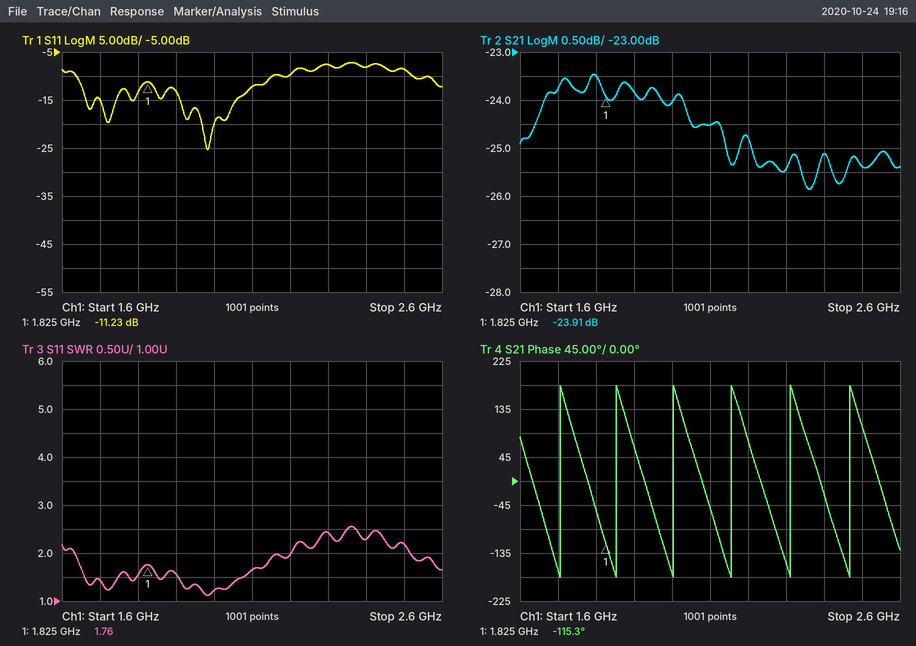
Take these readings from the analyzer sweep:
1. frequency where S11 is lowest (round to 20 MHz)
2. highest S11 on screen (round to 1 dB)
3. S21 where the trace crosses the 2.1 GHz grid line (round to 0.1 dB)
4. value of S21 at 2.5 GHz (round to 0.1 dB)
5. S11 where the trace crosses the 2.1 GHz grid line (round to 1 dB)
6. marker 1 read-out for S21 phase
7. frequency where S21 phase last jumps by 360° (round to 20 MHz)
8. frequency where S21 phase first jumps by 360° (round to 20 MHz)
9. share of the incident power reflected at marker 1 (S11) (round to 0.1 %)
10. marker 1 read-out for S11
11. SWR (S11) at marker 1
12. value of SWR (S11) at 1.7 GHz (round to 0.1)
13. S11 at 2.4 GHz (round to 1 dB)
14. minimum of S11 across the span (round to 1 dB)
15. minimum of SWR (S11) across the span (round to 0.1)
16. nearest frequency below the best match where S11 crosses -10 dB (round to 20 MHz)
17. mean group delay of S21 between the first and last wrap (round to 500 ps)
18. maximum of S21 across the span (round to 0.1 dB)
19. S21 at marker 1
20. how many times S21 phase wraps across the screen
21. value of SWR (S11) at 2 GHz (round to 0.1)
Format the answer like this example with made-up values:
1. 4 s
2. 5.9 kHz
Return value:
1. 1.98 GHz
2. -7 dB
3. -24.5 dB
4. -25.4 dB
5. -12 dB
6. -115.3°
7. 2.46 GHz
8. 1.70 GHz
9. 7.5 %
10. -11.23 dB
11. 1.76
12. 1.4
13. -8 dB
14. -25 dB
15. 1.1
16. 1.64 GHz
17. 6.5 ns
18. -23.5 dB
19. -23.91 dB
20. 6
21. 1.2
